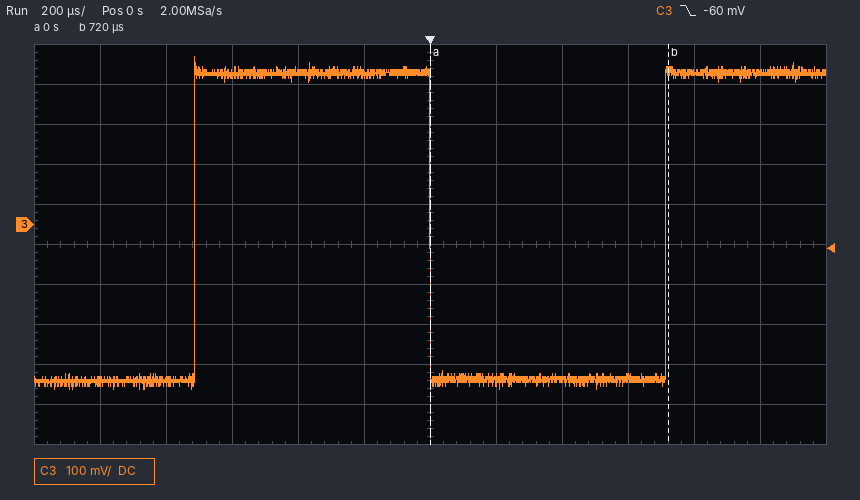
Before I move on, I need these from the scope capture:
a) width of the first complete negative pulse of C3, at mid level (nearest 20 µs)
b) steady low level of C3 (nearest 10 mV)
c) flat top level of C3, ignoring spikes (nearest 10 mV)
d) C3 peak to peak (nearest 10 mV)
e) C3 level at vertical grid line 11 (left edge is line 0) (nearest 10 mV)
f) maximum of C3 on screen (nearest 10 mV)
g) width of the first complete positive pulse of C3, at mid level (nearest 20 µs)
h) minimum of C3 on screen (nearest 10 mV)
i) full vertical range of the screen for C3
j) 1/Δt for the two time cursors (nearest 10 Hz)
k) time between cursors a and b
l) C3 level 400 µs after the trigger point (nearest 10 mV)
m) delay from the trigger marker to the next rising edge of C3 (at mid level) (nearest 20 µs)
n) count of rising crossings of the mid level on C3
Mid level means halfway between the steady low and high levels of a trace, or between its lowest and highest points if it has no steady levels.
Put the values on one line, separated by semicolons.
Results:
720 µs; -390 mV; 380 mV; 830 mV; 380 mV; 420 mV; 720 µs; -410 mV; 1 V; 1.39 kHz; 720 µs; -390 mV; 720 µs; 2
